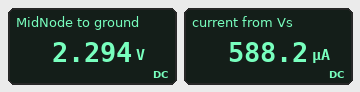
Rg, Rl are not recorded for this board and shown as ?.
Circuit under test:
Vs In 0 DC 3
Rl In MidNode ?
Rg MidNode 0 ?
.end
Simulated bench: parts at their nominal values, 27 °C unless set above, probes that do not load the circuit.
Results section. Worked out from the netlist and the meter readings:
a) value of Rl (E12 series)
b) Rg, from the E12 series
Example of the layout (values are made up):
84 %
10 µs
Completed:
1.2 kΩ
3.9 kΩ
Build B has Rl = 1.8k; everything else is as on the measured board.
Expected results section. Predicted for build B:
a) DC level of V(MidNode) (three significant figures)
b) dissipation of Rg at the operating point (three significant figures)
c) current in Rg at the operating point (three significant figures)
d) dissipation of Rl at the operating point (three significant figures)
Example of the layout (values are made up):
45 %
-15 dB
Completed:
2.05 V
1.08 mW
526 µA
499 µW
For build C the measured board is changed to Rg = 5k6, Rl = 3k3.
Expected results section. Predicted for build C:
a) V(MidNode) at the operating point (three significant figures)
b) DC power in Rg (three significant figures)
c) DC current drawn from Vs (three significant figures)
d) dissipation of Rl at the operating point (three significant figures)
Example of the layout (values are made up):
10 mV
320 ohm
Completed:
1.89 V
636 µW
337 µA
375 µW
